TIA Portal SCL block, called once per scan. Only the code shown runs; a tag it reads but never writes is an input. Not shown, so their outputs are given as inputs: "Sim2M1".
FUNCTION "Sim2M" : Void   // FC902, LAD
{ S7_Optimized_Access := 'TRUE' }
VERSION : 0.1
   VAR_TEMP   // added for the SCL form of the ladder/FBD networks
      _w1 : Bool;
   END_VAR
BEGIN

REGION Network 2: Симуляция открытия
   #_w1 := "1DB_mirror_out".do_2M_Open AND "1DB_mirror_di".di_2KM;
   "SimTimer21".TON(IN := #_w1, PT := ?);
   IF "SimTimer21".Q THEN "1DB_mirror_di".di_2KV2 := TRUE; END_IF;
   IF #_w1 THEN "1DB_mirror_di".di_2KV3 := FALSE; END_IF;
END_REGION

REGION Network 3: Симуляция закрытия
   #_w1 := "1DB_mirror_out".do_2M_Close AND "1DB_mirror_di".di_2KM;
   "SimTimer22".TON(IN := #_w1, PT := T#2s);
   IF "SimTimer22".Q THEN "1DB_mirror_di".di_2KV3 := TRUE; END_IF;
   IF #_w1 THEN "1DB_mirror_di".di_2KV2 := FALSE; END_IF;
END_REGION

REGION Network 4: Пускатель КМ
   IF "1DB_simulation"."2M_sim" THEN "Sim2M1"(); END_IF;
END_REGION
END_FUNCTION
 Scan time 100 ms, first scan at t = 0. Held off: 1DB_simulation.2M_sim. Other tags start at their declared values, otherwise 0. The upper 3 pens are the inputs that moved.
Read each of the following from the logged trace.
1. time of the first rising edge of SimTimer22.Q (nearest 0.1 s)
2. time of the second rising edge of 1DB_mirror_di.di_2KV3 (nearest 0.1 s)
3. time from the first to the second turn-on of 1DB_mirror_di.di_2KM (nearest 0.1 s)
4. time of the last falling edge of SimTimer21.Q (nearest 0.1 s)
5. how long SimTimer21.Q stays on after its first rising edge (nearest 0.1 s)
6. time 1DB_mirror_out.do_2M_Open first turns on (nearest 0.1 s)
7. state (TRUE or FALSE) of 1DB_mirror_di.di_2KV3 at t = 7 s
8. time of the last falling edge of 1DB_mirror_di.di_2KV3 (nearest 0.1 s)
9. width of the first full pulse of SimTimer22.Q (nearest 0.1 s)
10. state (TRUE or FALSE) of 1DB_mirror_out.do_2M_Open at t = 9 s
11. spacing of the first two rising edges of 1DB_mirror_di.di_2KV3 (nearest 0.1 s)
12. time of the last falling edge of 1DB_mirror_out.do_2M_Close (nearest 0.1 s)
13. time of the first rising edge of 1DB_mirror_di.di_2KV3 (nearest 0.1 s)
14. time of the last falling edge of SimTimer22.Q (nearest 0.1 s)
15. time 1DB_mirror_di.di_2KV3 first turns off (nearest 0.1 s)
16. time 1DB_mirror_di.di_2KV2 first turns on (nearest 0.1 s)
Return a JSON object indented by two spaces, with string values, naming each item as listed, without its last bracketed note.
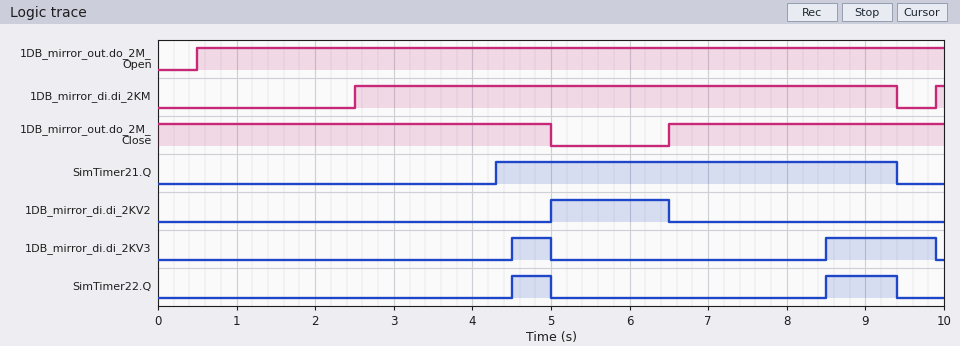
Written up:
{
  "time of the first rising edge of SimTimer22.Q": "4.5 s",
  "time of the second rising edge of 1DB_mirror_di.di_2KV3": "8.5 s",
  "time from the first to the second turn-on of 1DB_mirror_di.di_2KM": "7.4 s",
  "time of the last falling edge of SimTimer21.Q": "9.4 s",
  "how long SimTimer21.Q stays on after its first rising edge": "5.1 s",
  "time 1DB_mirror_out.do_2M_Open first turns on": "0.5 s",
  "state (TRUE or FALSE) of 1DB_mirror_di.di_2KV3 at t = 7 s": "FALSE",
  "time of the last falling edge of 1DB_mirror_di.di_2KV3": "9.9 s",
  "width of the first full pulse of SimTimer22.Q": "0.5 s",
  "state (TRUE or FALSE) of 1DB_mirror_out.do_2M_Open at t = 9 s": "TRUE",
  "spacing of the first two rising edges of 1DB_mirror_di.di_2KV3": "4.0 s",
  "time of the last falling edge of 1DB_mirror_out.do_2M_Close": "5.0 s",
  "time of the first rising edge of 1DB_mirror_di.di_2KV3": "4.5 s",
  "time of the last falling edge of SimTimer22.Q": "9.4 s",
  "time 1DB_mirror_di.di_2KV3 first turns off": "5.0 s",
  "time 1DB_mirror_di.di_2KV2 first turns on": "5.0 s"
}
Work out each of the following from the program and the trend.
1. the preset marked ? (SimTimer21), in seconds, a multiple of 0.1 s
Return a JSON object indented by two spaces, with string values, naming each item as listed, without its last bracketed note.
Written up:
{
  "the preset marked ? (SimTimer21), in seconds, a multiple of 0.1 s": "1.8 s"
}
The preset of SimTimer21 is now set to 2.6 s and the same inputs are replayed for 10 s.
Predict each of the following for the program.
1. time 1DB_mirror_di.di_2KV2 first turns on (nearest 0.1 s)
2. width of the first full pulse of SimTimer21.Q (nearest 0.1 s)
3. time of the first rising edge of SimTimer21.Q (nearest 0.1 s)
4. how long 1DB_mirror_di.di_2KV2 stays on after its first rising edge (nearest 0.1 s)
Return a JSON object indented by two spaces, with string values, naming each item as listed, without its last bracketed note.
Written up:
{
  "time 1DB_mirror_di.di_2KV2 first turns on": "5.1 s",
  "width of the first full pulse of SimTimer21.Q": "4.3 s",
  "time of the first rising edge of SimTimer21.Q": "5.1 s",
  "how long 1DB_mirror_di.di_2KV2 stays on after its first rising edge": "1.4 s"
}
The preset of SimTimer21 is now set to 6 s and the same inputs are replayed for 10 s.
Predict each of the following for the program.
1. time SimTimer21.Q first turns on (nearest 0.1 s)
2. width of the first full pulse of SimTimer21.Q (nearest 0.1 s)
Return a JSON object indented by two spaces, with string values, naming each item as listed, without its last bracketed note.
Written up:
{
  "time SimTimer21.Q first turns on": "8.5 s",
  "width of the first full pulse of SimTimer21.Q": "0.9 s"
}
